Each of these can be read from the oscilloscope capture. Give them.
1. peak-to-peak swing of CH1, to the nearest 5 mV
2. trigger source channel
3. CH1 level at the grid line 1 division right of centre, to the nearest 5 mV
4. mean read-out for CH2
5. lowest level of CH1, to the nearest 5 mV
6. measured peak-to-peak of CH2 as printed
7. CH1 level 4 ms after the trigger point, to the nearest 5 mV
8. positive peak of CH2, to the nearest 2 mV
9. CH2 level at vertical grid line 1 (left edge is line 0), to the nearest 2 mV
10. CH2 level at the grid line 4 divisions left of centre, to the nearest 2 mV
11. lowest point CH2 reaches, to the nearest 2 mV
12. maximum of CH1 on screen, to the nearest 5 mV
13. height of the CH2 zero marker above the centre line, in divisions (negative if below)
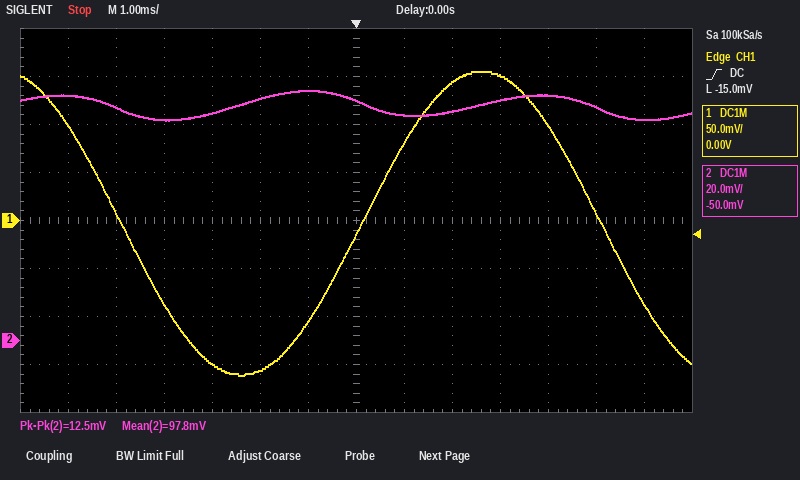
315 mV
CH1
80 mV
97.8 mV
-160 mV
12.5 mV
100 mV
104 mV
102 mV
92 mV
92 mV
155 mV
-2.5 div
